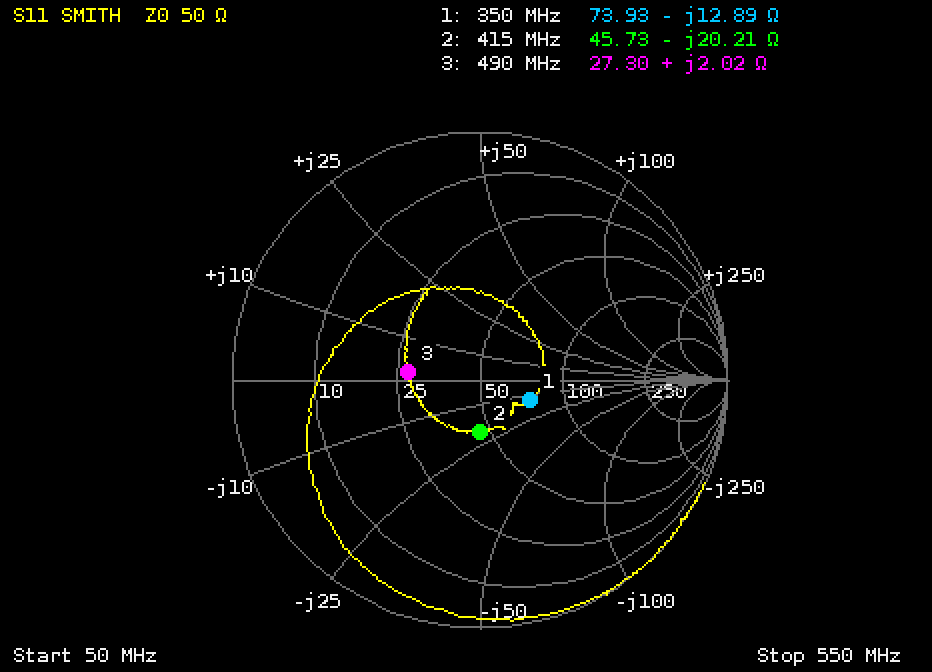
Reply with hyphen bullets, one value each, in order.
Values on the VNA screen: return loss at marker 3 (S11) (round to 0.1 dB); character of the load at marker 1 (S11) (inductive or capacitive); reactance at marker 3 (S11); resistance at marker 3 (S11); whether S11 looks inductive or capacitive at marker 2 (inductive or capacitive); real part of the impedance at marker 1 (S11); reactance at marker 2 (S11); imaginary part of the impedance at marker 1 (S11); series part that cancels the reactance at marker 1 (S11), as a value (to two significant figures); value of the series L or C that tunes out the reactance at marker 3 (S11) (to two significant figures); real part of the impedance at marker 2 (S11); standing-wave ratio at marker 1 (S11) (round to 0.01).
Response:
- 10.6 dB
- capacitive
- +2.02 Ω
- 27.30 Ω
- capacitive
- 73.93 Ω
- -20.21 Ω
- -12.89 Ω
- 5.9 nH
- 160 pF
- 45.73 Ω
- 1.56
